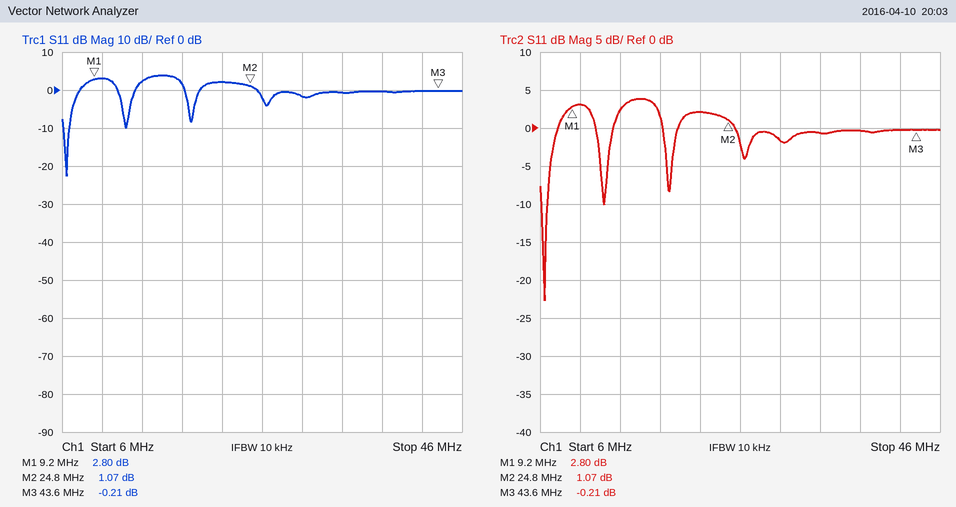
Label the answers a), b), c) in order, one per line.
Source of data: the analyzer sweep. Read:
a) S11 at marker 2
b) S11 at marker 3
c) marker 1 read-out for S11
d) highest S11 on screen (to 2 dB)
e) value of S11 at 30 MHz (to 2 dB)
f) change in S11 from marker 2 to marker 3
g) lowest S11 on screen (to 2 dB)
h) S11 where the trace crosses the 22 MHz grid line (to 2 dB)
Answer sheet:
a) 1.07 dB
b) -0.21 dB
c) 2.80 dB
d) 4 dB
e) -2 dB
f) -1.28 dB
g) -22 dB
h) 2 dB
